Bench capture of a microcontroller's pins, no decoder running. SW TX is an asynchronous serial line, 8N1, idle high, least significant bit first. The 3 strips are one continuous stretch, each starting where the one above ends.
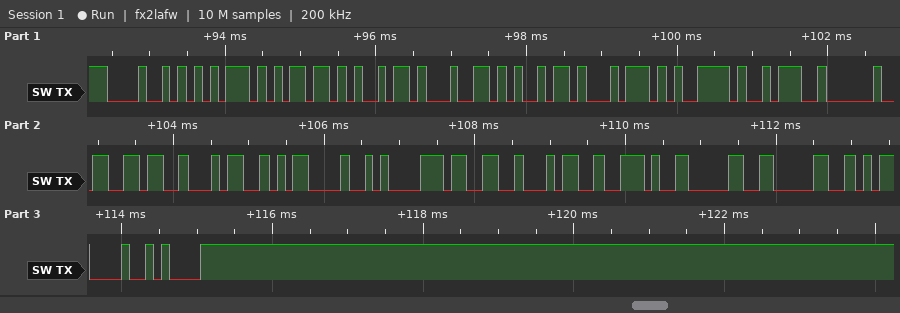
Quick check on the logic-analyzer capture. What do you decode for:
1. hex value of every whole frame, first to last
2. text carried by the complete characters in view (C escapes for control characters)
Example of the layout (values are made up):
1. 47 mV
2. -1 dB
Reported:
1. 48 75 6D 69 64 69 74 79 3A 20 36 34 0D 0A 33 34 2E 30 30 0D 0A
2. "Humidity: 64\r\n34.00\r\n"
